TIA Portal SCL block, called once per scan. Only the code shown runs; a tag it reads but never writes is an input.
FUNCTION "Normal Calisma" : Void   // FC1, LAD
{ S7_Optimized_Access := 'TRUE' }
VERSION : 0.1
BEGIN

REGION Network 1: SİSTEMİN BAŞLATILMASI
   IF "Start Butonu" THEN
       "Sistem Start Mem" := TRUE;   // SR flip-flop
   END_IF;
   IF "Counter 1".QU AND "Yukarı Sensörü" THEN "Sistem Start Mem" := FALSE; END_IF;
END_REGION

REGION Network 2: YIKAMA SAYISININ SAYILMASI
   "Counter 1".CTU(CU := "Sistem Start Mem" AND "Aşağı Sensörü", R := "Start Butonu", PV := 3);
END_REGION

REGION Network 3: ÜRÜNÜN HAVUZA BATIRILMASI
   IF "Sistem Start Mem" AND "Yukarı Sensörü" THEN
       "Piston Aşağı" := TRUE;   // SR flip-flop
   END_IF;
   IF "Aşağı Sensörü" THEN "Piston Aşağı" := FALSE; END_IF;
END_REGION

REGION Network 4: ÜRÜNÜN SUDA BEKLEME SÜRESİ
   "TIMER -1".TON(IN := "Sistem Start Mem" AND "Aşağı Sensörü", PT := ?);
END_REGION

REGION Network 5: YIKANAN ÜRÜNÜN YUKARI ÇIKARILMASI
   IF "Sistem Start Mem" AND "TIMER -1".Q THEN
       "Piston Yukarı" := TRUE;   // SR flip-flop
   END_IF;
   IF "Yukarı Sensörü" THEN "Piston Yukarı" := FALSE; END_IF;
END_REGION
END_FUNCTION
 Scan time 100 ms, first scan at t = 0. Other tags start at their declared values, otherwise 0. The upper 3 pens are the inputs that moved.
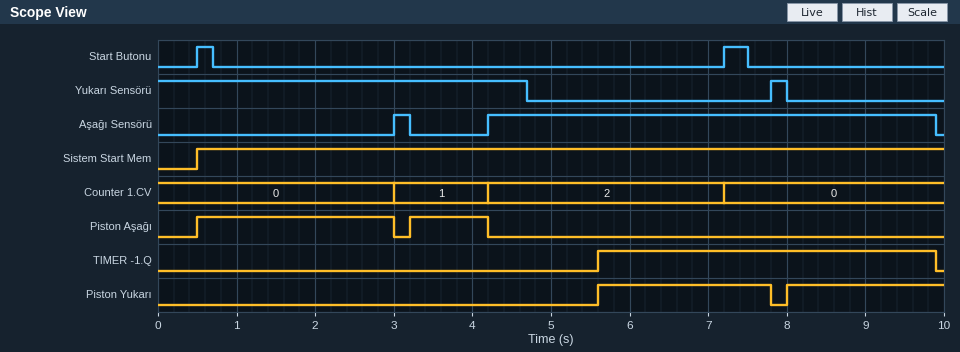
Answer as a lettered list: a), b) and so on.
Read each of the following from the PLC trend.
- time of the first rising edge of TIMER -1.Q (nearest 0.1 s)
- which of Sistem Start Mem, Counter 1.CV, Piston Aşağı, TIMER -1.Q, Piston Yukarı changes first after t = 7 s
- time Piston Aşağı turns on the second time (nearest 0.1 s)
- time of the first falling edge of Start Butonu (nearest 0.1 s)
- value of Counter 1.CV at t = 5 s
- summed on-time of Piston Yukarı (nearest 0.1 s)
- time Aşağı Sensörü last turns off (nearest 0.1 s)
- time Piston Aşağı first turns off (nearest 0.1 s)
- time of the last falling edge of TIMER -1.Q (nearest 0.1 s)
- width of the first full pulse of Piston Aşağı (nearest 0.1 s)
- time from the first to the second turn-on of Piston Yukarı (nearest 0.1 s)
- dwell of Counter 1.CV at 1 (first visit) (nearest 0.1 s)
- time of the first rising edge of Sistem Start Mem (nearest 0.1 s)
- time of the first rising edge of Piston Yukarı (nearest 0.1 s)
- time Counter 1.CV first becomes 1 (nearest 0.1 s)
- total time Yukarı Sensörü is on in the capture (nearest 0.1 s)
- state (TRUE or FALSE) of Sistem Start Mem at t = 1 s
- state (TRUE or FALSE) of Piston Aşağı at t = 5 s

a) 5.6 s
b) Counter 1.CV
c) 3.2 s
d) 0.7 s
e) 2
f) 4.2 s
g) 9.9 s
h) 3.0 s
i) 9.9 s
j) 2.5 s
k) 2.4 s
l) 1.2 s
m) 0.5 s
n) 5.6 s
o) 3.0 s
p) 4.9 s
q) TRUE
r) FALSE
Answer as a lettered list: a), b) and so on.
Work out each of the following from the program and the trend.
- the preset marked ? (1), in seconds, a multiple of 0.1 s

a) 1.4 s
